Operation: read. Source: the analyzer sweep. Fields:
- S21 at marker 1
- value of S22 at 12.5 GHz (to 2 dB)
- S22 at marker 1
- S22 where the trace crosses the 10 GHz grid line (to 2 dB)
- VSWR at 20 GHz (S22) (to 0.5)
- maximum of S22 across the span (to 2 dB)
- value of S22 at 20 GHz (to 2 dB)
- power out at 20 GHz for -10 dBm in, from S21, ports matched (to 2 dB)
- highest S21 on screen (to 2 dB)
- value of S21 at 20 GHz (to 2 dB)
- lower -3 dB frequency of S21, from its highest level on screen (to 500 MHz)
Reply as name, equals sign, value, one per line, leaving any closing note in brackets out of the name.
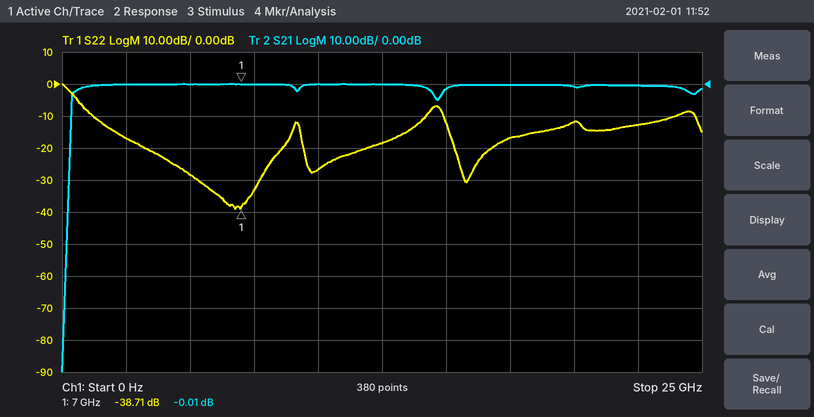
S21 at marker 1 = -0.01 dB
value of S22 at 12.5 GHz = -18 dB
S22 at marker 1 = -38.71 dB
S22 where the trace crosses the 10 GHz grid line = -26 dB
VSWR at 20 GHz (S22) = 1.5
maximum of S22 across the span = 0 dB
value of S22 at 20 GHz = -12 dB
power out at 20 GHz for -10 dBm in, from S21, ports matched = -10 dBm
highest S21 on screen = 0 dB
value of S21 at 20 GHz = 0 dB
lower -3 dB frequency of S21, from its highest level on screen = 500 MHz
